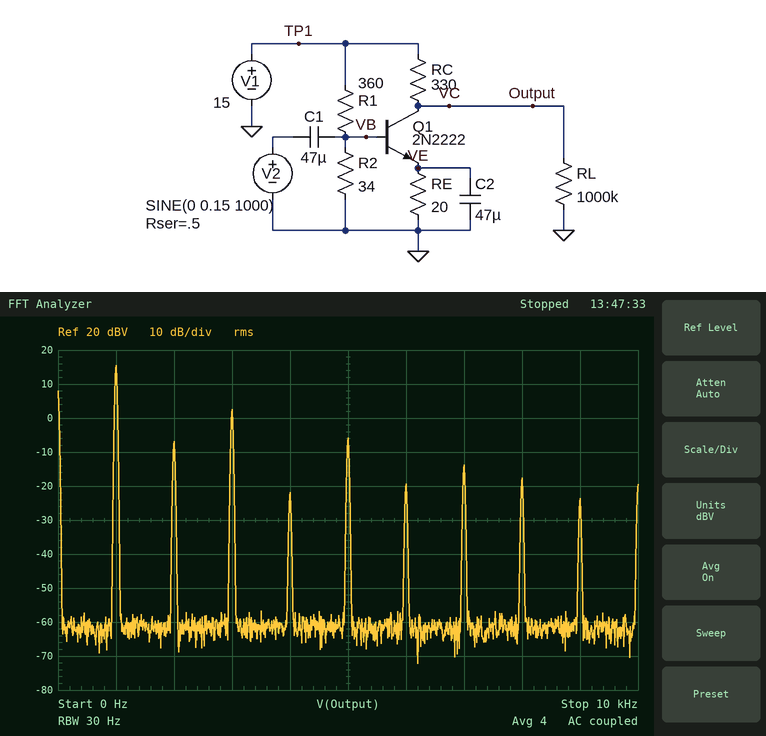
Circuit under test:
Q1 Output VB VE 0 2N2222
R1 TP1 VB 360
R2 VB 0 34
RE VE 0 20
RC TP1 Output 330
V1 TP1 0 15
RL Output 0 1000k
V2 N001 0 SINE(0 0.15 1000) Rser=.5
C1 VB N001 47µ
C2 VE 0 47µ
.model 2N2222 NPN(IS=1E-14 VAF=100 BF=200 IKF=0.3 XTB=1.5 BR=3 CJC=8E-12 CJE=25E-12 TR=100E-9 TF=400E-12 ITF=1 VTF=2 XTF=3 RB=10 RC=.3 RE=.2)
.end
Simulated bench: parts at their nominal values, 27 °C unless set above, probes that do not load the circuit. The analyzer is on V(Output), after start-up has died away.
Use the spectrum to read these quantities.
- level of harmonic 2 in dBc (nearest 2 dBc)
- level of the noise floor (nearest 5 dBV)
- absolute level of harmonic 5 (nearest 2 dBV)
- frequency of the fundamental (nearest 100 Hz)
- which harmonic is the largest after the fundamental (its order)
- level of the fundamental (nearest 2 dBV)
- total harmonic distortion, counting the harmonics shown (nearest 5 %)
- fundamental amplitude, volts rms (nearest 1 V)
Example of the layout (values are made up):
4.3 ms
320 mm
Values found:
-22 dBc
-60 dBV
-6 dBV
1.0 kHz
3
16 dBV
25 %
6 V
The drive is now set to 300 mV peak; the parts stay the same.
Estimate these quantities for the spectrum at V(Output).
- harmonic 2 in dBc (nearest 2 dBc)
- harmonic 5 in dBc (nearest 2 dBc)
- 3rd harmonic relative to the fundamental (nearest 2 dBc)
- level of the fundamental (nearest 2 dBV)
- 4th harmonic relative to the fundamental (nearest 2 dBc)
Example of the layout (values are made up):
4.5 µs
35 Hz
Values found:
-18 dBc
-18 dBc
-10 dBc
16 dBV
-20 dBc
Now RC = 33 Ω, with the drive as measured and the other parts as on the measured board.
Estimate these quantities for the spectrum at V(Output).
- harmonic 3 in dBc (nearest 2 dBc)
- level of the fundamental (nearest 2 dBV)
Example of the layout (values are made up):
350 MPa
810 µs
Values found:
-22 dBc
-2 dBV
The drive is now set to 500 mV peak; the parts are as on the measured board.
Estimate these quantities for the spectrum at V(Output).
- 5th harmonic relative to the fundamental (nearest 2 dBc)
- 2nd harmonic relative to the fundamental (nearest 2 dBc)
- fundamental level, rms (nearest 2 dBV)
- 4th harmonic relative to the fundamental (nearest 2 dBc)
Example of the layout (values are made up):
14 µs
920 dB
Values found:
-24 dBc
-12 dBc
16 dBV
-14 dBc
